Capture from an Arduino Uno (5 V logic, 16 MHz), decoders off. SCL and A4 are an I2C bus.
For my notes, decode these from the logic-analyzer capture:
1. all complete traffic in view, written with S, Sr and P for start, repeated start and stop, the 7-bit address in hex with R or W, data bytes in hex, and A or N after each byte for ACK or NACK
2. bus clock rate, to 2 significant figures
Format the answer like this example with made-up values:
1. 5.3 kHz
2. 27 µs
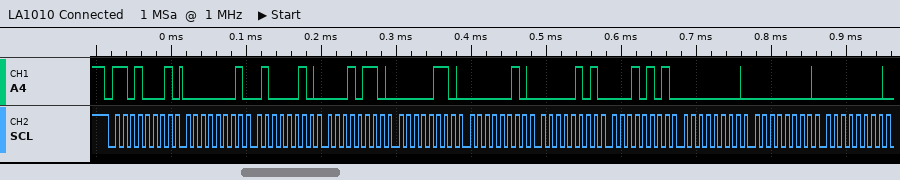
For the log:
1. S 68R A 01 A 42 A 16 A 06 A 02 A 05 A 15 A 00 A 00 A 00 A
2. 100 kHz
